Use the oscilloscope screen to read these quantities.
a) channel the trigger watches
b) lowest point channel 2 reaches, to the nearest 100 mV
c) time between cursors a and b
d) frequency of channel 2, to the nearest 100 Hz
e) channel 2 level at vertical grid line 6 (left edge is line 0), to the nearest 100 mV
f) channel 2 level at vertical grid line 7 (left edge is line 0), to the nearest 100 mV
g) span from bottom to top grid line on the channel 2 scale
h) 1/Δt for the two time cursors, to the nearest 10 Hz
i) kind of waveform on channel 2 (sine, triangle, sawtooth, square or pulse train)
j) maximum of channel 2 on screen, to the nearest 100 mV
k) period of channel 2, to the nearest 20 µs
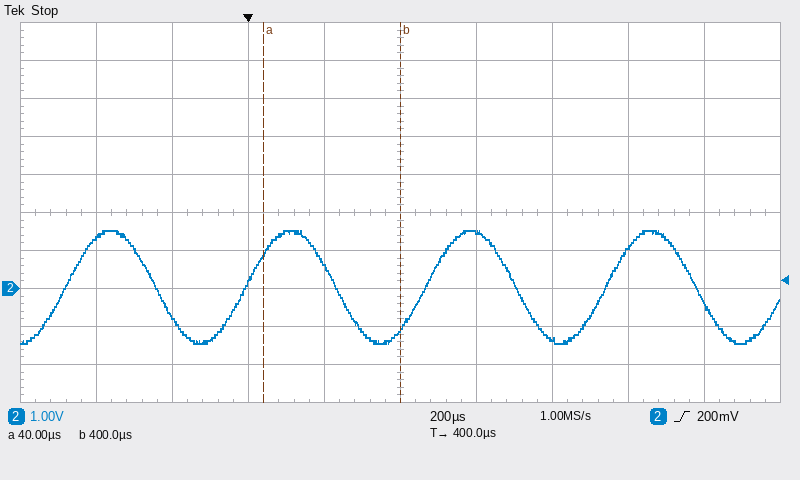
channel 2
-1.4 V
360 µs
2.1 kHz
1.5 V
-1.4 V
10 V
2.78 kHz
sine
1.5 V
480 µs
